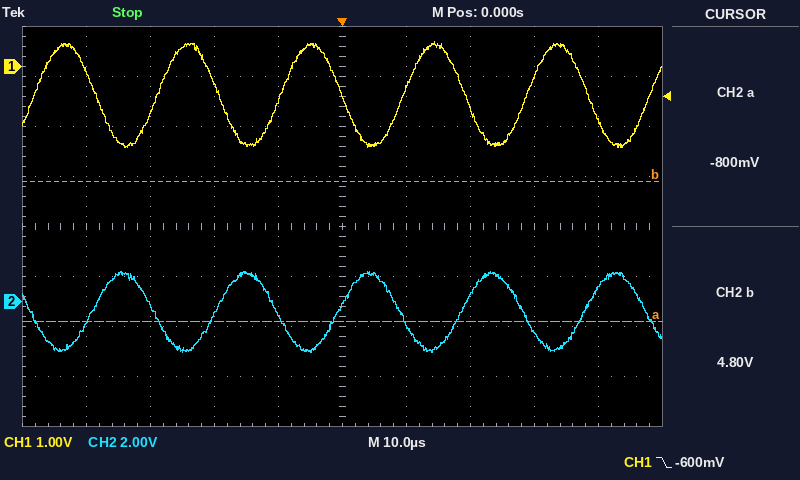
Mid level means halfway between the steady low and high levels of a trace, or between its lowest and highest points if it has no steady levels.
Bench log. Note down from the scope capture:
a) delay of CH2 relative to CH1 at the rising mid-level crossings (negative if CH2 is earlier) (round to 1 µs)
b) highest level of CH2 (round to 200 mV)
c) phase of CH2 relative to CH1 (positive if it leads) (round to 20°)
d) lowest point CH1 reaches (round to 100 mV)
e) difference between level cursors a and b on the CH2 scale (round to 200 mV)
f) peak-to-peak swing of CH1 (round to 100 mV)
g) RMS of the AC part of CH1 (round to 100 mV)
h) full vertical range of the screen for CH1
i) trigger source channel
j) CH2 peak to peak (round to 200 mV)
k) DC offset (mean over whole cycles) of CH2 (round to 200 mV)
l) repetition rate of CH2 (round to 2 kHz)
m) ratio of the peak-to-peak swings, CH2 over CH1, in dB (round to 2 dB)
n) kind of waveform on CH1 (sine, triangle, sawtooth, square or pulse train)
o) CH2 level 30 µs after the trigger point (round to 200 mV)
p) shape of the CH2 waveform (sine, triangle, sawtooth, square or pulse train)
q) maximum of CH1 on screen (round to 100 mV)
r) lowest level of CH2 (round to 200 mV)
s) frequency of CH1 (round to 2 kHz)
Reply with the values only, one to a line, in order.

+9 µs
1.2 V
-160°
-1.6 V
5.6 V
2.1 V
700 mV
8 V
CH1
3.2 V
-400 mV
52 kHz
4 dB
sine
-1.2 V
sine
500 mV
-2.0 V
52 kHz
